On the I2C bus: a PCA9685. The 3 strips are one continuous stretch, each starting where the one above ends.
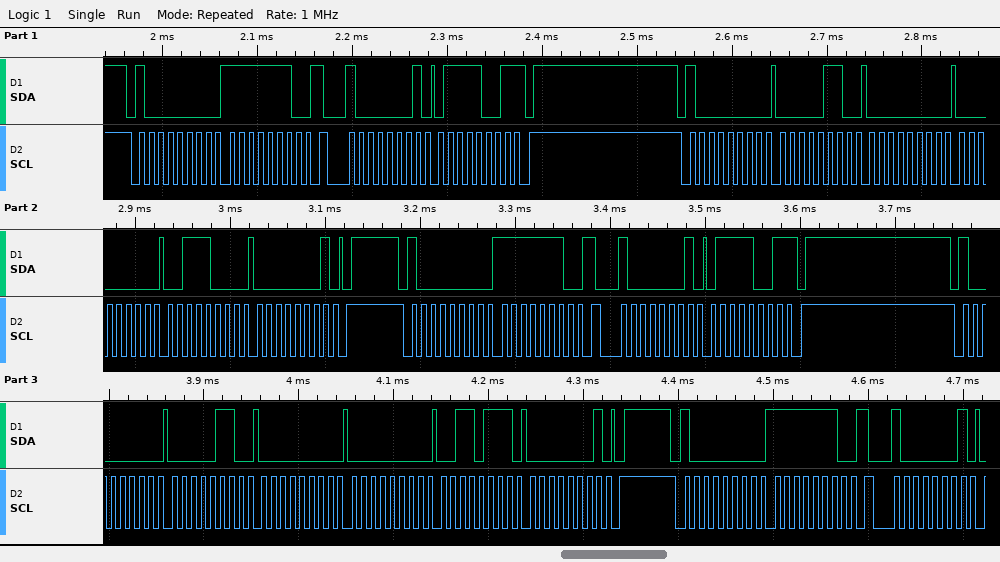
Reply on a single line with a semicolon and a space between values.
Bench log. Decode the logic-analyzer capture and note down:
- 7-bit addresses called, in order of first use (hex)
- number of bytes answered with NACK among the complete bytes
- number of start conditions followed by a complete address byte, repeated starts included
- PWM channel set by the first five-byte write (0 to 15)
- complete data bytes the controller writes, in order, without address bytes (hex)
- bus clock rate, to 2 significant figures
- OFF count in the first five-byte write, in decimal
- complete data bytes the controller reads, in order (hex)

0x40; 2; 8; 0; FE 06 00 00 38 01 FE 06 00 00 37 01 FE; 100 kHz; 312; 79 79
